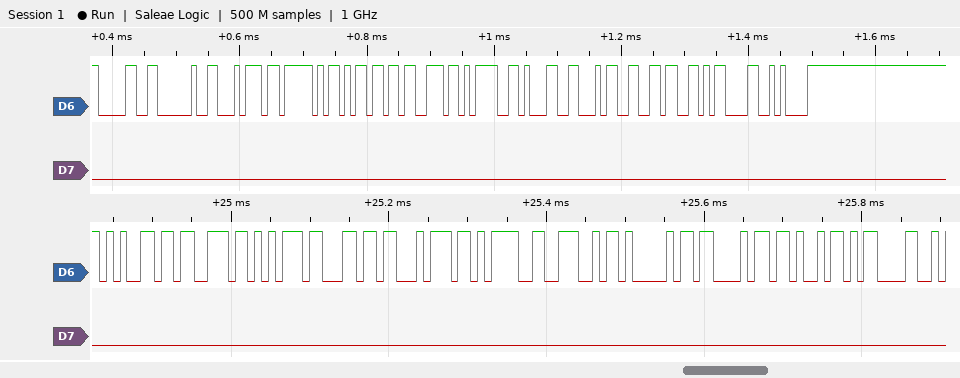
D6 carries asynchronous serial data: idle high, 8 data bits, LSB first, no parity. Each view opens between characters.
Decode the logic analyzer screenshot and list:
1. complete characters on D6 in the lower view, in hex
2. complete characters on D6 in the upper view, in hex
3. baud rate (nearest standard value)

65, 73, 75, 6C, 74, 3D, 4E, 41, 43, 4B, 0D
30, 20, 74, 5F, 6D, 73, 3D, 31, 34, 36, 0D, 0A
115200 baud
